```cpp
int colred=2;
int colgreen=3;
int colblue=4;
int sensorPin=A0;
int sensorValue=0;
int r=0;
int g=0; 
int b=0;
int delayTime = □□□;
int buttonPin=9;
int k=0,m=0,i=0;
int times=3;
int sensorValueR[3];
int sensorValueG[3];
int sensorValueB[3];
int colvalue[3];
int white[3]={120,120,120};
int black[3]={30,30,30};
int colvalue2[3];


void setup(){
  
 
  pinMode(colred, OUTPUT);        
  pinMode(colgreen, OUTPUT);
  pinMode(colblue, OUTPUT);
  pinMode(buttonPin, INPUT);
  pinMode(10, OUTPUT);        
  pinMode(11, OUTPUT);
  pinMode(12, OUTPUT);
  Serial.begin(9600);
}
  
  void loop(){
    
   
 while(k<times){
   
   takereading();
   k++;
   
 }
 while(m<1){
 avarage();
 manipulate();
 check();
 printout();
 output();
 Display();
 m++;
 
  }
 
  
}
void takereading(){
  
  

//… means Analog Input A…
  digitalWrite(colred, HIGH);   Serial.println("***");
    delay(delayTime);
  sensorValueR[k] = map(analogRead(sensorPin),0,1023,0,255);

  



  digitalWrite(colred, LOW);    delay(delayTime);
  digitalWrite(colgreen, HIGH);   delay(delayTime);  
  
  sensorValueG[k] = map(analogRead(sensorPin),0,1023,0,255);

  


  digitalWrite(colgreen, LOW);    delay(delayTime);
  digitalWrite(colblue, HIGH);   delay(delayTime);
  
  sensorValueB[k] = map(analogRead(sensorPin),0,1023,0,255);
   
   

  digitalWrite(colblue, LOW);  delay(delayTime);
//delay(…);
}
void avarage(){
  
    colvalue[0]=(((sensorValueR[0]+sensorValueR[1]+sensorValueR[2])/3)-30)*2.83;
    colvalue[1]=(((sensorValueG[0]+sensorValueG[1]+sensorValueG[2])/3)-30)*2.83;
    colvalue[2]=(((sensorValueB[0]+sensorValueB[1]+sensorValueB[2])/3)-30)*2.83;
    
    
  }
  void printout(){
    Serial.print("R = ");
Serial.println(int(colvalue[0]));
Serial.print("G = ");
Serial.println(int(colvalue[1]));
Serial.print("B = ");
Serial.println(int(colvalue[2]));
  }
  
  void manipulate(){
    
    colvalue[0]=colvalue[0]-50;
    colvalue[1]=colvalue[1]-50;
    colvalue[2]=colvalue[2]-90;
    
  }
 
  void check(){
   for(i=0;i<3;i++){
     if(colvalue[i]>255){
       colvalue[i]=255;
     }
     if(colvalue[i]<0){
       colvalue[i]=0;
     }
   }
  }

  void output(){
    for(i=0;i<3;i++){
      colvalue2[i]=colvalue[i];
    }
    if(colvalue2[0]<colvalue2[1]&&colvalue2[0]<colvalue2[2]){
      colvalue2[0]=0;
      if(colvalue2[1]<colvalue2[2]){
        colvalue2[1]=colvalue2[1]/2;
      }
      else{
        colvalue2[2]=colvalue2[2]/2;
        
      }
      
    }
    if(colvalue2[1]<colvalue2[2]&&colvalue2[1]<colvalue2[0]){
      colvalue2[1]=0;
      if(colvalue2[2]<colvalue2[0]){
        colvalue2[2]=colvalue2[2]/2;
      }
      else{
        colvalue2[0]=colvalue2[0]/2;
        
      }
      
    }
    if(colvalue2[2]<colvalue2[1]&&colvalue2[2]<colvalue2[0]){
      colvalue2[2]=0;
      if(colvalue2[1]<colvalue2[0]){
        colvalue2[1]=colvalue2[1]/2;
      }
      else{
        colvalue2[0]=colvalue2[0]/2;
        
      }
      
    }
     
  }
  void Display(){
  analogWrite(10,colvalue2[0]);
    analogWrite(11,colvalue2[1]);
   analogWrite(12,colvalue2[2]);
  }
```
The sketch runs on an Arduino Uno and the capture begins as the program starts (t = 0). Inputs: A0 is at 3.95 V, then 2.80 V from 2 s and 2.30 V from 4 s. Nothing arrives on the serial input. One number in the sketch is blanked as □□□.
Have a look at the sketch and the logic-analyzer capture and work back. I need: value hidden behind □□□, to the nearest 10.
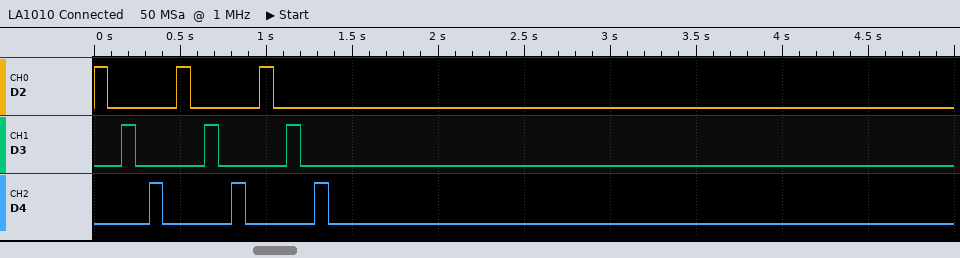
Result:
80
